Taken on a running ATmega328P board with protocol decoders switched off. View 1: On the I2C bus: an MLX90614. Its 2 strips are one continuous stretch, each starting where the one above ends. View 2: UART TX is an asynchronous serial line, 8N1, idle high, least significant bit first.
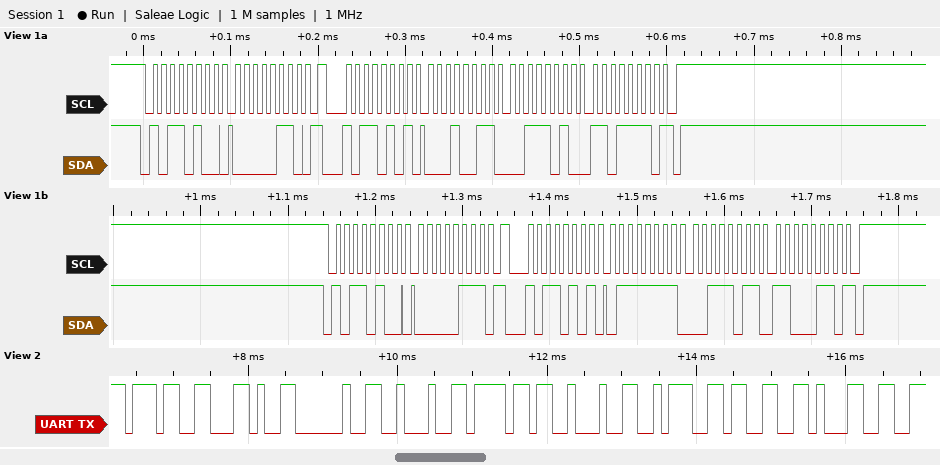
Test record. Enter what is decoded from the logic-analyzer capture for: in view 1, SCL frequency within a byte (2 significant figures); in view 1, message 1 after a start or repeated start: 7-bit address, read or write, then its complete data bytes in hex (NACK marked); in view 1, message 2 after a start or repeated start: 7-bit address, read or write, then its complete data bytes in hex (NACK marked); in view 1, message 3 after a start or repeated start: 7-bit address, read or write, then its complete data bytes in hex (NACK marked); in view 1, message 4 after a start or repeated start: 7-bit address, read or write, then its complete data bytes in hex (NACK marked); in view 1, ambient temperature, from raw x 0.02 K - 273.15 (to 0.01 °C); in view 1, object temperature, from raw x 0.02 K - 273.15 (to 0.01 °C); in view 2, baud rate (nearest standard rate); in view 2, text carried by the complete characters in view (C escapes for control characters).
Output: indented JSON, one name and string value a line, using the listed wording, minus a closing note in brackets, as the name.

{
  "in view 1, SCL frequency within a byte": "100 kHz",
  "in view 1, message 1 after a start or repeated start: 7-bit address, read or write, then its complete data bytes in hex": "0x5A write: 06",
  "in view 1, message 2 after a start or repeated start: 7-bit address, read or write, then its complete data bytes in hex": "0x5A read: 13 3A DE NACK",
  "in view 1, message 3 after a start or repeated start: 7-bit address, read or write, then its complete data bytes in hex": "0x5A write: 07",
  "in view 1, message 4 after a start or repeated start: 7-bit address, read or write, then its complete data bytes in hex": "0x5A read: 7F 3B C6 NACK",
  "in view 1, ambient temperature, from raw x 0.02 K - 273.15": "24.19 °C",
  "in view 1, object temperature, from raw x 0.02 K - 273.15": "31.47 °C",
  "in view 2, baud rate": "9600 baud",
  "in view 2, text carried by the complete characters in view": "\"7, \\\"o\\\":31\""
}
